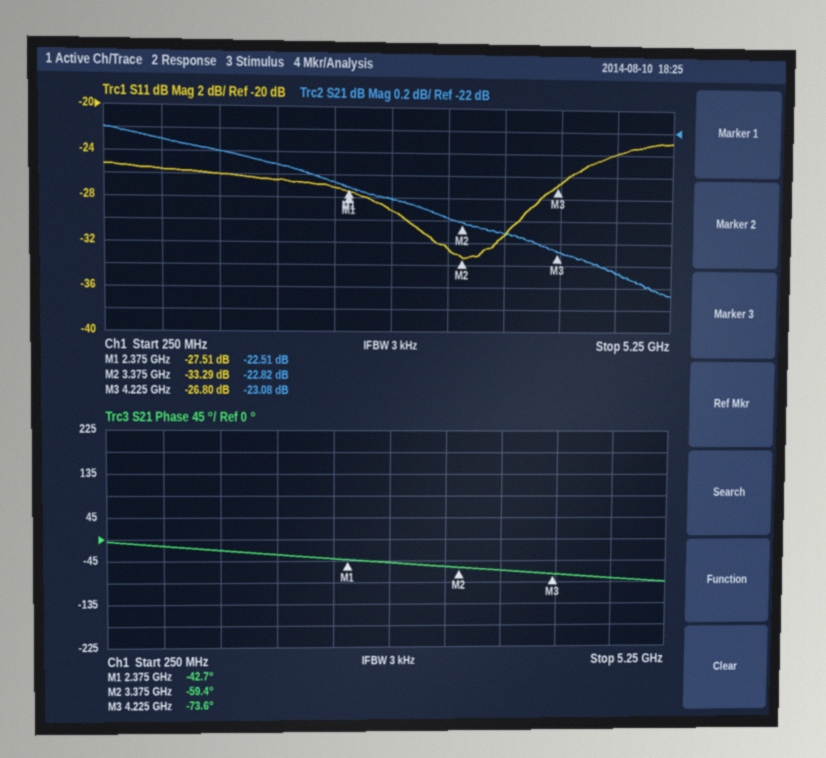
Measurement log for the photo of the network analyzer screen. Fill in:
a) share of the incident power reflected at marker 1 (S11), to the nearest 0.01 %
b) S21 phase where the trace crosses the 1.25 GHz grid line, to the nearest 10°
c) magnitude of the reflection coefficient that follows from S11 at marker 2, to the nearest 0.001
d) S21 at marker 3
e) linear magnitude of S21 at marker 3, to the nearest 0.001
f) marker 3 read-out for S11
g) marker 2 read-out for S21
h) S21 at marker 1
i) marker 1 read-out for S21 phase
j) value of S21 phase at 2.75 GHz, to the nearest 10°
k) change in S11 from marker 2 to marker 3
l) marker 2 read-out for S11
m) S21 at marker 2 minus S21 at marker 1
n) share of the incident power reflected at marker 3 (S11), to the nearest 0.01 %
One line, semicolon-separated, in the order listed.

0.18 %; -20°; 0.022; -23.08 dB; 0.070; -26.80 dB; -22.82 dB; -22.51 dB; -42.7°; -50°; 6.49 dB; -33.29 dB; -0.31 dB; 0.21 %
